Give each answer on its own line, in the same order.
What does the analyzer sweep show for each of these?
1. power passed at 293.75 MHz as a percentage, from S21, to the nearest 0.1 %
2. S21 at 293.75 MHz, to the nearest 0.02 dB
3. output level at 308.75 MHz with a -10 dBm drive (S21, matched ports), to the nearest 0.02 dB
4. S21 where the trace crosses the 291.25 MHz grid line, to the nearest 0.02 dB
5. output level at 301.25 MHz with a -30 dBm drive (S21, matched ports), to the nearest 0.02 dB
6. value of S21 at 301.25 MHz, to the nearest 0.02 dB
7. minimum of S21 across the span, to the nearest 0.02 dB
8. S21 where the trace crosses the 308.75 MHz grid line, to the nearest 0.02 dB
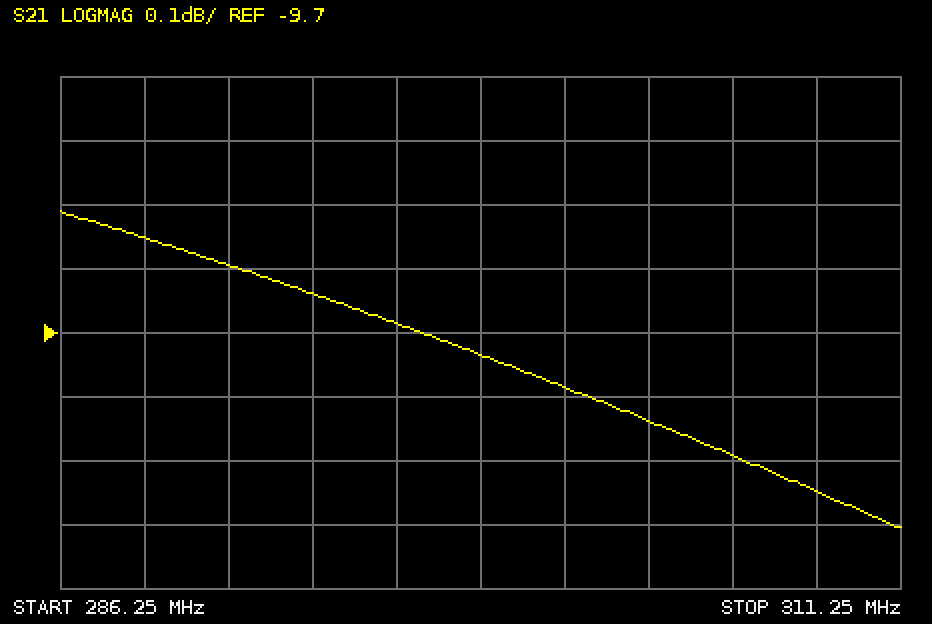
10.9 %
-9.64 dB
-19.94 dBm
-9.60 dB
-39.78 dBm
-9.78 dB
-10.00 dB
-9.94 dB
